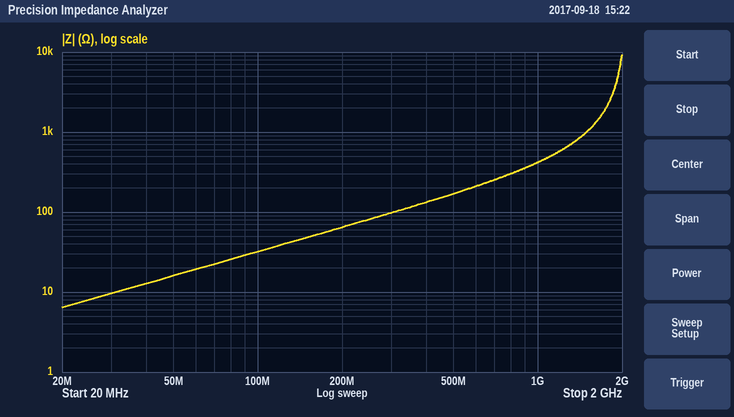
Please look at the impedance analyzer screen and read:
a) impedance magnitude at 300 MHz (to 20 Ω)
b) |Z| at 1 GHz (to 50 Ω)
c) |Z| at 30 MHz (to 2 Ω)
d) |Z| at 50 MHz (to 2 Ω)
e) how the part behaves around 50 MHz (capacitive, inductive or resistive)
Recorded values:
100 Ω
400 Ω
10 Ω
16 Ω
inductive
